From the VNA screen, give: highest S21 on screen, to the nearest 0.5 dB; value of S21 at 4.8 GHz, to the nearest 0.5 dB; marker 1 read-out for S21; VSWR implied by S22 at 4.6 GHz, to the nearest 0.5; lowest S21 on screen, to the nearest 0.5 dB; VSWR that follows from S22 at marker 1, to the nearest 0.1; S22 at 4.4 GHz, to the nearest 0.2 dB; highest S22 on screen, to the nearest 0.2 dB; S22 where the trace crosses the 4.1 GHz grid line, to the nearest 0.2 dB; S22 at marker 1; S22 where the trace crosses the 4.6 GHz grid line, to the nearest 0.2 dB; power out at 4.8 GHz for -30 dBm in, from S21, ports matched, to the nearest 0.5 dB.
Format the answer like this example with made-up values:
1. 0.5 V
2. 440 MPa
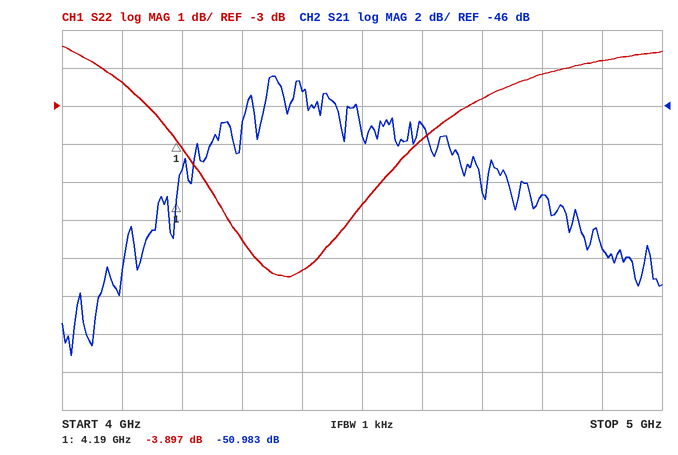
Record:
1. -44.5 dB
2. -50.5 dB
3. -50.983 dB
4. 4.5
5. -59.0 dB
6. 4.5
7. -7.4 dB
8. -1.4 dB
9. -2.4 dB
10. -3.897 dB
11. -3.8 dB
12. -80.5 dBm
